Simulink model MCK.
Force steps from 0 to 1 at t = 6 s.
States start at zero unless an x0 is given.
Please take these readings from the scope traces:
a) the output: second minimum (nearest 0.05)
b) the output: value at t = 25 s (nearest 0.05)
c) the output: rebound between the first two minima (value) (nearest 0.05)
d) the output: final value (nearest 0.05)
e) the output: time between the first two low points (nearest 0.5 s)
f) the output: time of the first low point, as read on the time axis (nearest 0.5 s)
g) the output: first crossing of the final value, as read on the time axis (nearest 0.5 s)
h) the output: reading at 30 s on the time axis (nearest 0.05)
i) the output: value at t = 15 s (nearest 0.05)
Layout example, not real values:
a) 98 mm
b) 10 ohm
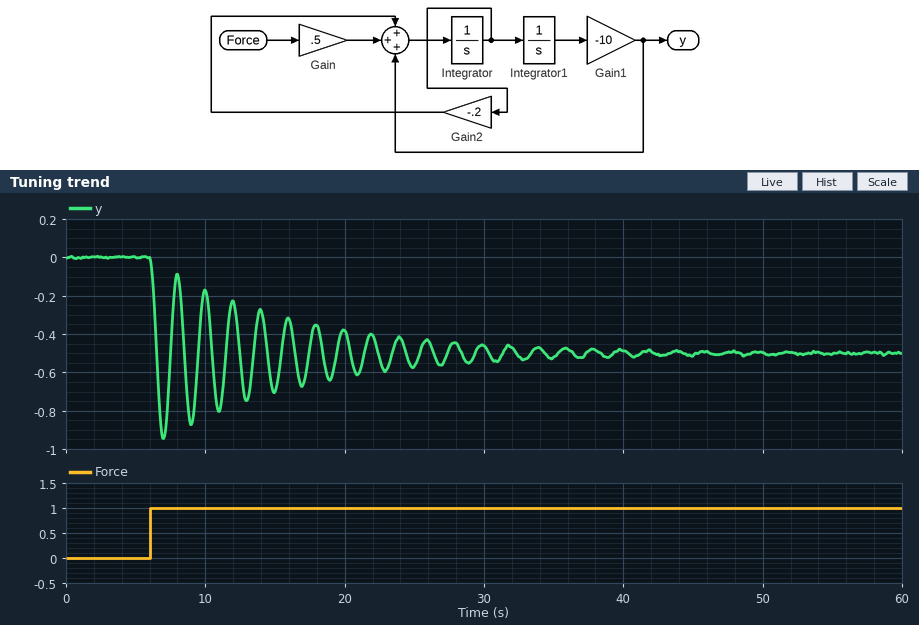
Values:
a) -0.85
b) -0.55
c) -0.10
d) -0.50
e) 2.0 s
f) 7.0 s
g) 6.5 s
h) -0.45
i) -0.70
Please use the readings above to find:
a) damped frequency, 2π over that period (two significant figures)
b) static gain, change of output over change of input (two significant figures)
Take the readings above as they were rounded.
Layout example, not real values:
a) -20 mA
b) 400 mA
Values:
a) 3.1 rad/s
b) -0.50
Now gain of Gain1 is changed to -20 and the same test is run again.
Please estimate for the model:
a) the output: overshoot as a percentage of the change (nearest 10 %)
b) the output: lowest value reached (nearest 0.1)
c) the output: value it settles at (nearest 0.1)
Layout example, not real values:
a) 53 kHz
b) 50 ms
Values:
a) 90 %
b) -1.0
c) -0.5
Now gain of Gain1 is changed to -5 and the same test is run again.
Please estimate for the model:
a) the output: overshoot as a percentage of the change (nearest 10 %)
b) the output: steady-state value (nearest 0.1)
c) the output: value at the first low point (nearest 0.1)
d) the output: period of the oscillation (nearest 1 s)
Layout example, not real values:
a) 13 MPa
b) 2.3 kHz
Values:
a) 90 %
b) -0.5
c) -0.9
d) 3 s
